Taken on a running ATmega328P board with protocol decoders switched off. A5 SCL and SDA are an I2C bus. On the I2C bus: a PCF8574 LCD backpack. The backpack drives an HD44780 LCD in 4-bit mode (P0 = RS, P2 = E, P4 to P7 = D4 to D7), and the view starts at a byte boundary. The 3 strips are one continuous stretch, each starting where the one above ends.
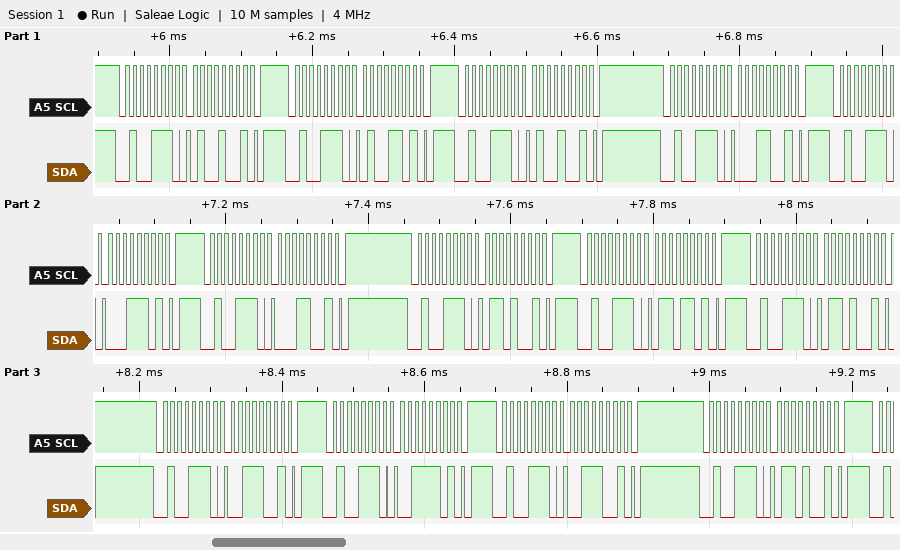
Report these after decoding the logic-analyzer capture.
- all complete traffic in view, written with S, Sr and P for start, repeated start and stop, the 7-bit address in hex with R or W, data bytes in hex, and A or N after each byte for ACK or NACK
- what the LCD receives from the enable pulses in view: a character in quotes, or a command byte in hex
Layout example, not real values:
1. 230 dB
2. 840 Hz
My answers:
1. S 27W A 49 A P S 27W A 4D A P S 27W A 49 A P S 27W A 19 A P S 27W A 1D A P S 27W A 19 A P S 27W A 69 A P S 27W A 6D A P S 27W A 69 A P S 27W A 39 A P S 27W A 3D A P S 27W A 39 A P S 27W A 69 A P
2. 'A' 'c'
